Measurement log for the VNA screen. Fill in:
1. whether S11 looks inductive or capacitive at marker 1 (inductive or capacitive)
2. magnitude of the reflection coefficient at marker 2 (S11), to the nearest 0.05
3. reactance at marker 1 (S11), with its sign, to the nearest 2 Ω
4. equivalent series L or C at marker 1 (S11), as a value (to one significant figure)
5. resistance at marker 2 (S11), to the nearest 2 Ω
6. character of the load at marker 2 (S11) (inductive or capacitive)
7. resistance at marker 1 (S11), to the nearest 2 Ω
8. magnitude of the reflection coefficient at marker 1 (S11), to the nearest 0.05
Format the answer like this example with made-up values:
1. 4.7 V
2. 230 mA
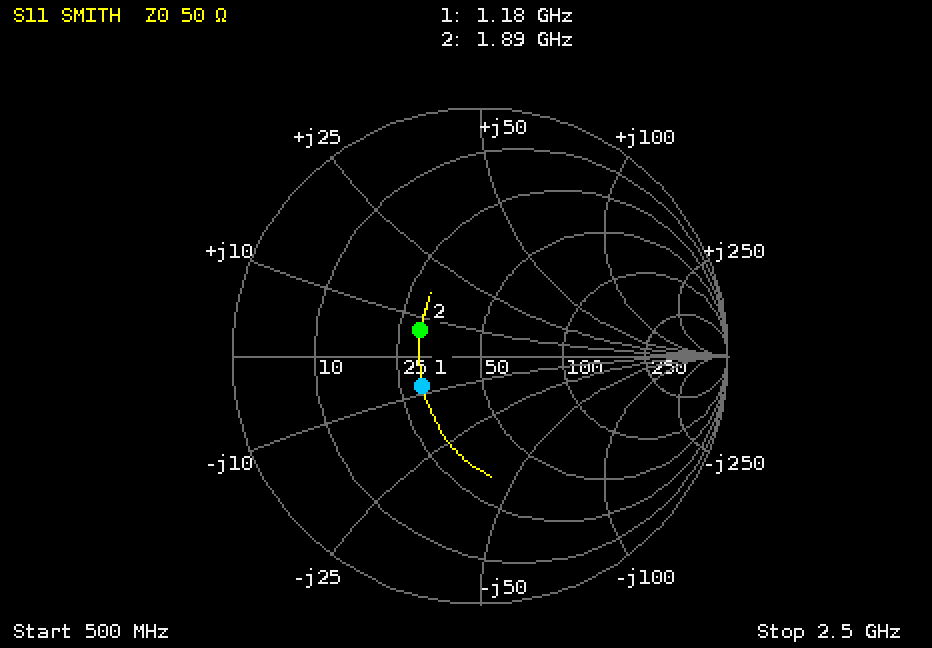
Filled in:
1. capacitive
2. 0.25
3. -8 Ω
4. 20 pF
5. 30 Ω
6. inductive
7. 30 Ω
8. 0.25
